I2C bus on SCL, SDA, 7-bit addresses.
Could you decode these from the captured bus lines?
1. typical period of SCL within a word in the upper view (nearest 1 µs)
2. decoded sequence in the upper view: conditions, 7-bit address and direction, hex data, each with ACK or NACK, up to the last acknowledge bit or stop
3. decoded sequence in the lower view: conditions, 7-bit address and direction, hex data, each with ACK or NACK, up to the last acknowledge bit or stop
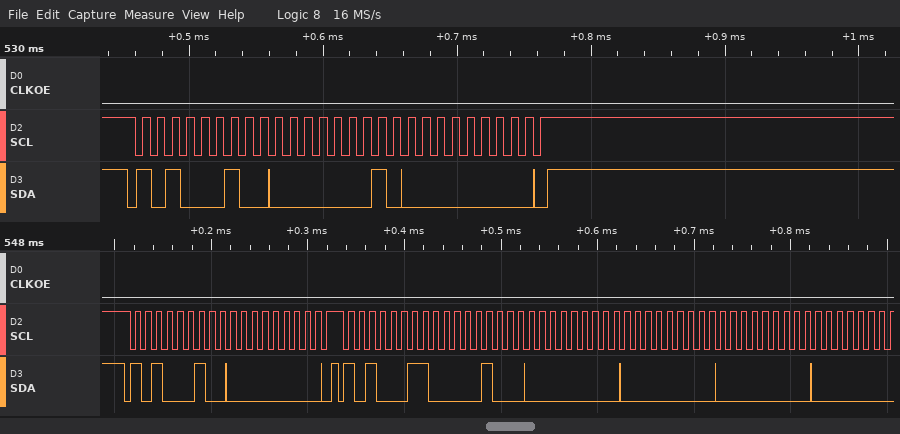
11 µs
start, address 51 write ACK, 01 ACK, 00 ACK, stop
start, address 51 write ACK, 00 ACK, stop, start, address 51 read ACK, 08 ACK, 00 ACK, 00 ACK, 00 ACK
